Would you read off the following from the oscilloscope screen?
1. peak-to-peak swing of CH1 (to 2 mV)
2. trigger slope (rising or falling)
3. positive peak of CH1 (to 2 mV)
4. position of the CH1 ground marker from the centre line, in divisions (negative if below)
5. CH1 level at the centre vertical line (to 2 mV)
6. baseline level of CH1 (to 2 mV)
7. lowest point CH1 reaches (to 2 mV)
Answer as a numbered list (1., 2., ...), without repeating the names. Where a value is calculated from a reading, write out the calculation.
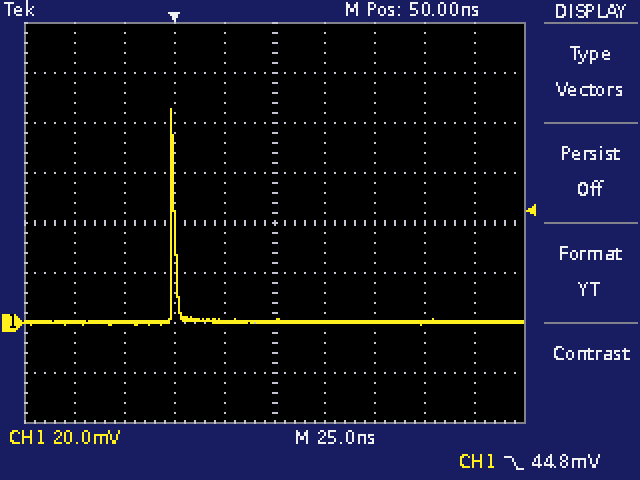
1. 86 mV − (0 mV) = 86 mV
2. falling
3. 86 mV
4. -2.0 div
5. 0 mV
6. 0 mV
7. 0 mV
